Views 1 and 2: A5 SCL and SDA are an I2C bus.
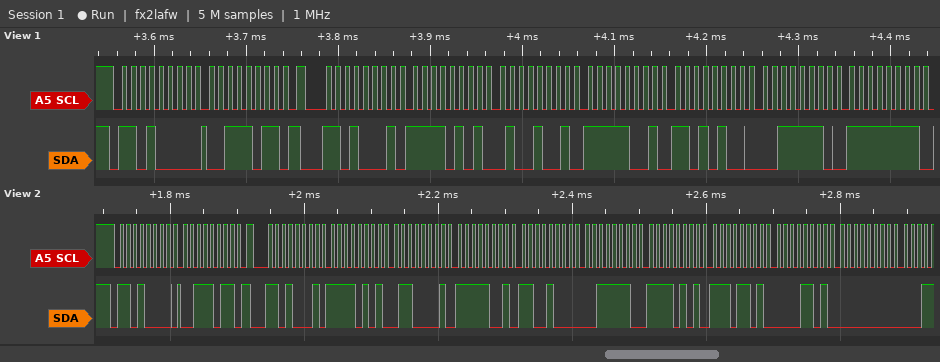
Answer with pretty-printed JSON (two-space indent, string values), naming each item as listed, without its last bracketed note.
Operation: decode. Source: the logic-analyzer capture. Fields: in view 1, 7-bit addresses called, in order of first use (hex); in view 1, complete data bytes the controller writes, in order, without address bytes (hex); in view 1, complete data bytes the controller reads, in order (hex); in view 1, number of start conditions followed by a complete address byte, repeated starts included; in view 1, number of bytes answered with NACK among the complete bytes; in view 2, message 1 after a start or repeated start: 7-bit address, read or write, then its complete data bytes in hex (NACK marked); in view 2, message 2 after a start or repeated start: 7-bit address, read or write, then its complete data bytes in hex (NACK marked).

{
  "in view 1, 7-bit addresses called, in order of first use": "0x68",
  "in view 1, complete data bytes the controller writes, in order, without address bytes": "3B",
  "in view 1, complete data bytes the controller reads, in order": "F5 49 F9 D4 3E FF",
  "in view 1, number of start conditions followed by a complete address byte, repeated starts included": "2",
  "in view 1, number of bytes answered with NACK among the complete bytes": "0",
  "in view 2, message 1 after a start or repeated start: 7-bit address, read or write, then its complete data bytes in hex": "0x68 write: 3B",
  "in view 2, message 2 after a start or repeated start: 7-bit address, read or write, then its complete data bytes in hex": "0x68 read: F5 61 F9 C8 3E F5 ED 0D 00"
}
